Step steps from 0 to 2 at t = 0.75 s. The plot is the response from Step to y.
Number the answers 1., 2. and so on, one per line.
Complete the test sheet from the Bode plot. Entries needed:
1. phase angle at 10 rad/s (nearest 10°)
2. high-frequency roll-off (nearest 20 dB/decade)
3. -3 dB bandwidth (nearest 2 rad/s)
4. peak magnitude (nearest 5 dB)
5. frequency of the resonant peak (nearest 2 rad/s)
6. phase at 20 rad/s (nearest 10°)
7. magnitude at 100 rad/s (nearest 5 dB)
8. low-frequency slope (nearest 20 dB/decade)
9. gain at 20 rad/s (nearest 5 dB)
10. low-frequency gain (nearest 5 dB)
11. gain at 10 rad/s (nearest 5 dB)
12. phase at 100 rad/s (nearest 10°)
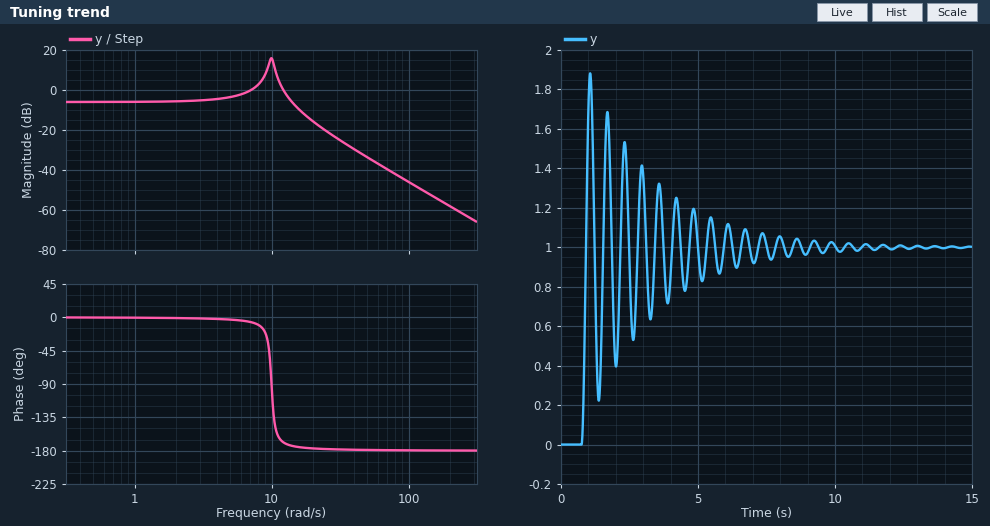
1. -90°
2. -40 dB/decade
3. 16 rad/s
4. 15 dB
5. 10 rad/s
6. -180°
7. -45 dB
8. 0 dB/decade
9. -15 dB
10. -5 dB
11. 15 dB
12. -180°
